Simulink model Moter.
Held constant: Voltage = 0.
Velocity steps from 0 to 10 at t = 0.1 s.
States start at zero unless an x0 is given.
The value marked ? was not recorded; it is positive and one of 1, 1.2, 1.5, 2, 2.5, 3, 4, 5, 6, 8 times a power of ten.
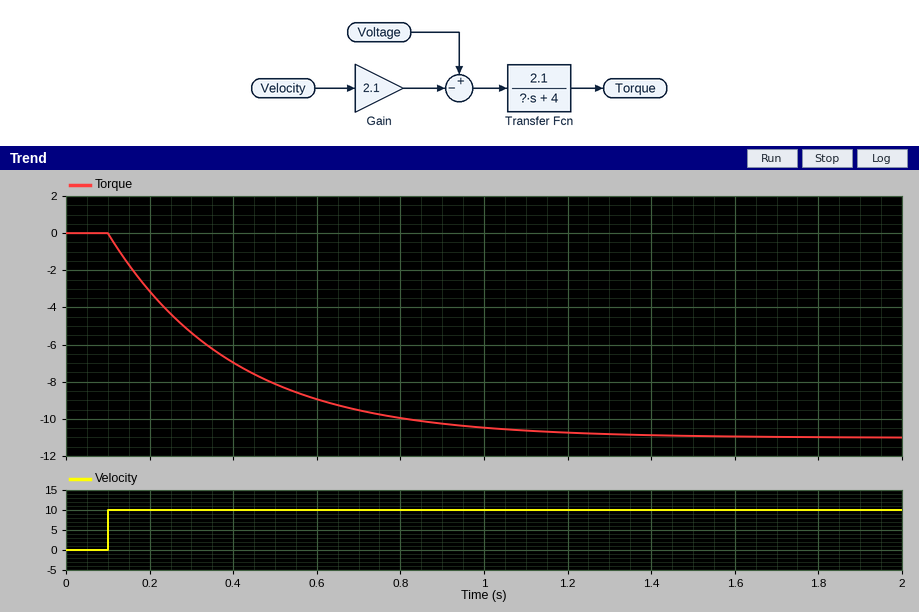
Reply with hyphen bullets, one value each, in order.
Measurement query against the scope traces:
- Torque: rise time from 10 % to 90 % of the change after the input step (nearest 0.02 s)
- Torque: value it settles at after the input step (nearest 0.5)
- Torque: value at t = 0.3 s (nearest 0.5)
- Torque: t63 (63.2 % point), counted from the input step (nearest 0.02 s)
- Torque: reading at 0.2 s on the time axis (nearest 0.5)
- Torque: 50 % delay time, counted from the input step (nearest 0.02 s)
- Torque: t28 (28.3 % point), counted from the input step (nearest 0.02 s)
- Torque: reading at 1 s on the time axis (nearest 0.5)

- 0.66 s
- -11.0
- -5.5
- 0.30 s
- -3.0
- 0.20 s
- 0.10 s
- -10.5
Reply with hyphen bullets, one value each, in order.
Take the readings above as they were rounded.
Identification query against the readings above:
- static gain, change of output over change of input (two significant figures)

- -1.1
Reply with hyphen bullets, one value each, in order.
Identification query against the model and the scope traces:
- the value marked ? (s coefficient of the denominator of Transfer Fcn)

- 1.2
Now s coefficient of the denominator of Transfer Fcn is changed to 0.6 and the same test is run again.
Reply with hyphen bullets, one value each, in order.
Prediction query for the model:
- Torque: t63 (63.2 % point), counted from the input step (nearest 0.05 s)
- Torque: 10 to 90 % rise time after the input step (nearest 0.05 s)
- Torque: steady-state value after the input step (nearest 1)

- 0.15 s
- 0.35 s
- -11
